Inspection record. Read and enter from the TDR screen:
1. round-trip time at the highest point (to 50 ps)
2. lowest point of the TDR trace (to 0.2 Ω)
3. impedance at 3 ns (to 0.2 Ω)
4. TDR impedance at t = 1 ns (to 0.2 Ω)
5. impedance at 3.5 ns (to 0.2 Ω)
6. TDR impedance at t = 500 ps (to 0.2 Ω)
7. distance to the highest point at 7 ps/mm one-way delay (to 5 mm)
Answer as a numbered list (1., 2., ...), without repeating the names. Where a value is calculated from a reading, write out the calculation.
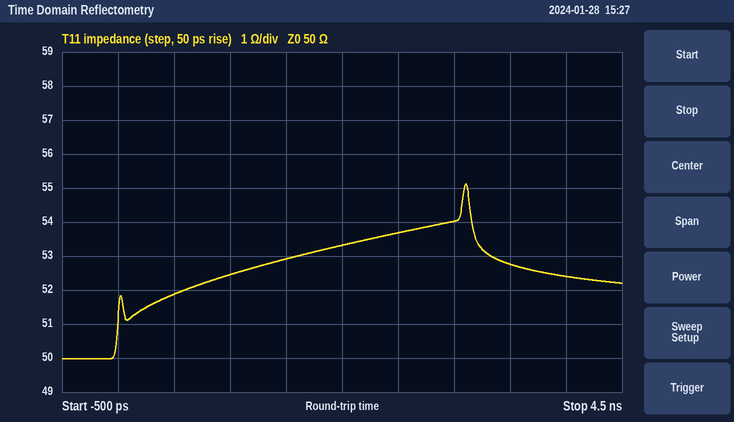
1. 3.10 ns
2. 50.0 Ω
3. 54.0 Ω
4. 52.4 Ω
5. 52.8 Ω
6. 51.8 Ω
7. 3.10 ns / 2 / 7 ps/mm ≈ 221 mm, so 220 mm to the nearest 5 mm
